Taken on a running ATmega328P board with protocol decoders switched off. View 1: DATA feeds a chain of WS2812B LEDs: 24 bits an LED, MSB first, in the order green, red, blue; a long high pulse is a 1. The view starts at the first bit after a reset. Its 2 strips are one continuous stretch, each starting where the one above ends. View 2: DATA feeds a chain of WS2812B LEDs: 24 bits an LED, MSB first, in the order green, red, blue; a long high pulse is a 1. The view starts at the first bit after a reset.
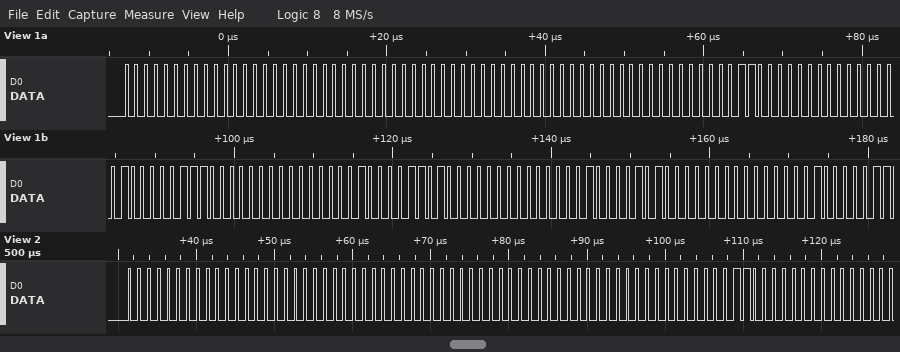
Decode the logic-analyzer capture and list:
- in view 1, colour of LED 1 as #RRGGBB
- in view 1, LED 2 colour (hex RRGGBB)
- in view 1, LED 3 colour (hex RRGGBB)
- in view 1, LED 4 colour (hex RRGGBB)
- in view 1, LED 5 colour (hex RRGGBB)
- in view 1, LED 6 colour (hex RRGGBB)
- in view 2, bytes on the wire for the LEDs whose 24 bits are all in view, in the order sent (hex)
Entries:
#000000
#000000
#030000
#070100
#0D0100
#140200
00 00 00 00 00 00 00 03 00
